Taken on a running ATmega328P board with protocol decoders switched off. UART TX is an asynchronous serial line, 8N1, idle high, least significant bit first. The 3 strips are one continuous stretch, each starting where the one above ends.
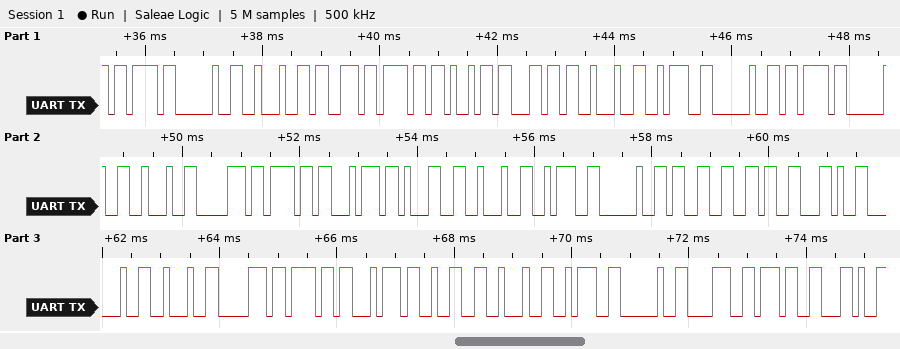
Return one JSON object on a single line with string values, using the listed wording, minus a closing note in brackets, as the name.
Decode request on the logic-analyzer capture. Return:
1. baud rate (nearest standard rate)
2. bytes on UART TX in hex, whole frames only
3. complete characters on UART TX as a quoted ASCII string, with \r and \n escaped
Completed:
{"baud rate": "9600 baud", "bytes on UART TX in hex, whole frames only": "7B 20 22 73 6F 69 6C 22 3A 20 7B 20 22 70 6F 74 31 22 3A 20 33 36 2C 20 22 70 6F 74 32 22 3A 20 38 37 2C", "complete characters on UART TX as a quoted ASCII string, with \\r and \\n escaped": "\"{ \\\"soil\\\": { \\\"pot1\\\": 36, \\\"pot2\\\": 87,\""}
